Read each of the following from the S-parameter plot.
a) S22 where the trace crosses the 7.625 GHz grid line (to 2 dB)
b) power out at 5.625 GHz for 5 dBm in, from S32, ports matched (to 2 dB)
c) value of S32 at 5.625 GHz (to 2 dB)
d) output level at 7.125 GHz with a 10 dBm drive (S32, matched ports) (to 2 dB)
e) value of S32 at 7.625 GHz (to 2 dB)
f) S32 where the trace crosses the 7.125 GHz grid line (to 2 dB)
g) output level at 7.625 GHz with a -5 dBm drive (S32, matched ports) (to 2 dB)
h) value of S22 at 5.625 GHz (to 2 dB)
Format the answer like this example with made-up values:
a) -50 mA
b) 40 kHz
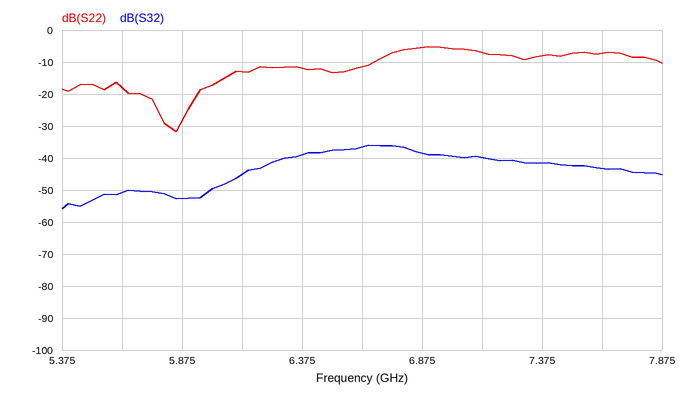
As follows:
a) -8 dB
b) -46 dBm
c) -50 dB
d) -30 dBm
e) -44 dB
f) -40 dB
g) -48 dBm
h) -18 dB
